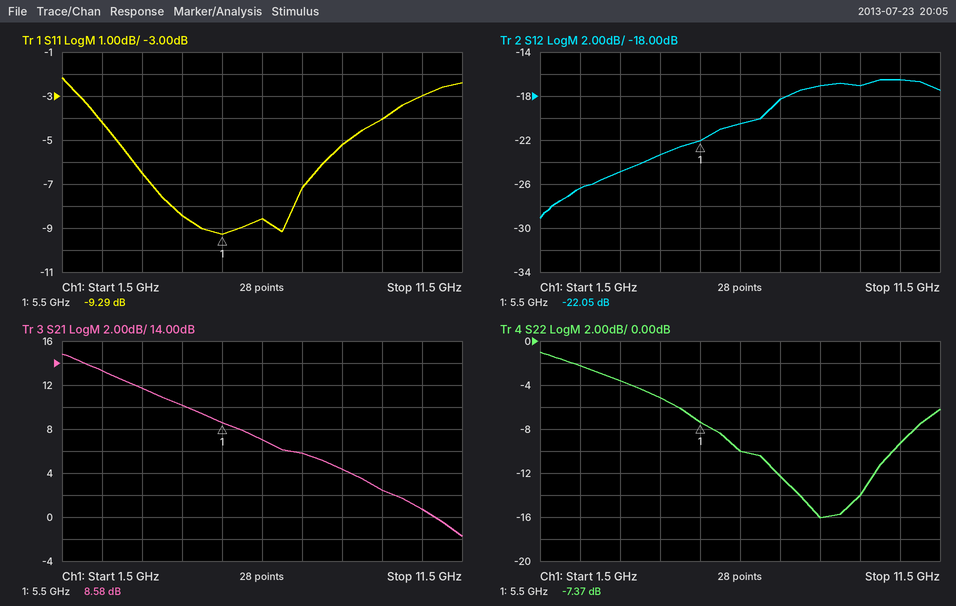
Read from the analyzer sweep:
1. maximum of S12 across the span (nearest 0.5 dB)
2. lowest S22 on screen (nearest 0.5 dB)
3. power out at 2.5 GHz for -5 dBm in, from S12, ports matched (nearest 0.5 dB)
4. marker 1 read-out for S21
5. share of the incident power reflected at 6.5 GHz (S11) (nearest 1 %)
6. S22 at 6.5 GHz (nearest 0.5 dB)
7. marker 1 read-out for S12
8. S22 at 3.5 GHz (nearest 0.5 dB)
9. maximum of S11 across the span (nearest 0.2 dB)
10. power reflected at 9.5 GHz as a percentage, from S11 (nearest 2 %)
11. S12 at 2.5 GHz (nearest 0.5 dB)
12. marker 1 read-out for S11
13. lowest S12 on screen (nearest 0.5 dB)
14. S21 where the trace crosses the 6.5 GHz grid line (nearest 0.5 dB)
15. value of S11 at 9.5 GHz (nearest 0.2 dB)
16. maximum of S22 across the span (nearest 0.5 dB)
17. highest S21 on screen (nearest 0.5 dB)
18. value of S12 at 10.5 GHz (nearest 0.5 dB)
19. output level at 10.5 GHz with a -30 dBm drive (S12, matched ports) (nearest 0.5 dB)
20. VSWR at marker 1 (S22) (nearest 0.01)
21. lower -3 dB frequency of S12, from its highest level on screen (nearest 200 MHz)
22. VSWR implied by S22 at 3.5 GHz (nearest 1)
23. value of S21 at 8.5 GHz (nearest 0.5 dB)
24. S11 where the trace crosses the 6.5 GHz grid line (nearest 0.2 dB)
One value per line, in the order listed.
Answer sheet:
-16.5 dB
-16.0 dB
-31.5 dBm
8.58 dB
14 %
-10.0 dB
-22.05 dB
-3.5 dB
-2.2 dB
40 %
-26.5 dB
-9.29 dB
-29.0 dB
7.0 dB
-4.0 dB
-1.0 dB
15.0 dB
-16.5 dB
-46.5 dBm
2.50
7.2 GHz
5
4.5 dB
-8.6 dB
